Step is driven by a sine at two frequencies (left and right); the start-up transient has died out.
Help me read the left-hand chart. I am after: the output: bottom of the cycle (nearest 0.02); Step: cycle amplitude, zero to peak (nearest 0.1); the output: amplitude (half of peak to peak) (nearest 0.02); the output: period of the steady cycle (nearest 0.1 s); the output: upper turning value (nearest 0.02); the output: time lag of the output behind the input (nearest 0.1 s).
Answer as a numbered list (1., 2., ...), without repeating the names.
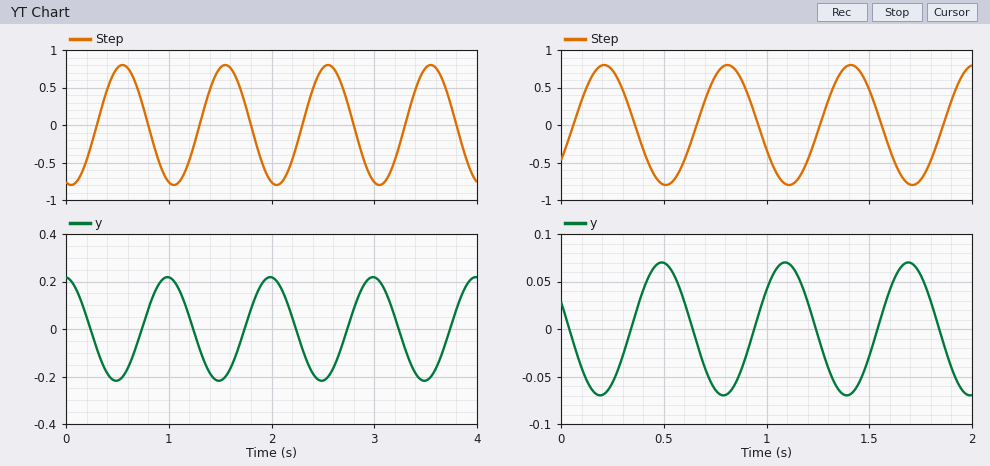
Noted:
1. -0.22
2. 0.8
3. 0.22
4. 1.0 s
5. 0.22
6. 0.4 s
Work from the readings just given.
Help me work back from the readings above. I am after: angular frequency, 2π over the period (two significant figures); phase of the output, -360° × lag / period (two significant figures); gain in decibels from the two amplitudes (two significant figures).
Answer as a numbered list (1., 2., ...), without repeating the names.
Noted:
1. 6.3 rad/s
2. -140°
3. -11 dB
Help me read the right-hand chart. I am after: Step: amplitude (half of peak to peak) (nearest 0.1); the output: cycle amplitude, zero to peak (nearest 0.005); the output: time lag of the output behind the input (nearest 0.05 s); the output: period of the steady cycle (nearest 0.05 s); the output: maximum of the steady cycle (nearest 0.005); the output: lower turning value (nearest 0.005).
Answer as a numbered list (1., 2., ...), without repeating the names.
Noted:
1. 0.8
2. 0.070
3. 0.30 s
4. 0.60 s
5. 0.070
6. -0.070
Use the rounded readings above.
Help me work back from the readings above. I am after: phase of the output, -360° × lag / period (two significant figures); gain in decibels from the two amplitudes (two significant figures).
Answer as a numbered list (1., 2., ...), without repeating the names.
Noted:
1. -180°
2. -21 dB
